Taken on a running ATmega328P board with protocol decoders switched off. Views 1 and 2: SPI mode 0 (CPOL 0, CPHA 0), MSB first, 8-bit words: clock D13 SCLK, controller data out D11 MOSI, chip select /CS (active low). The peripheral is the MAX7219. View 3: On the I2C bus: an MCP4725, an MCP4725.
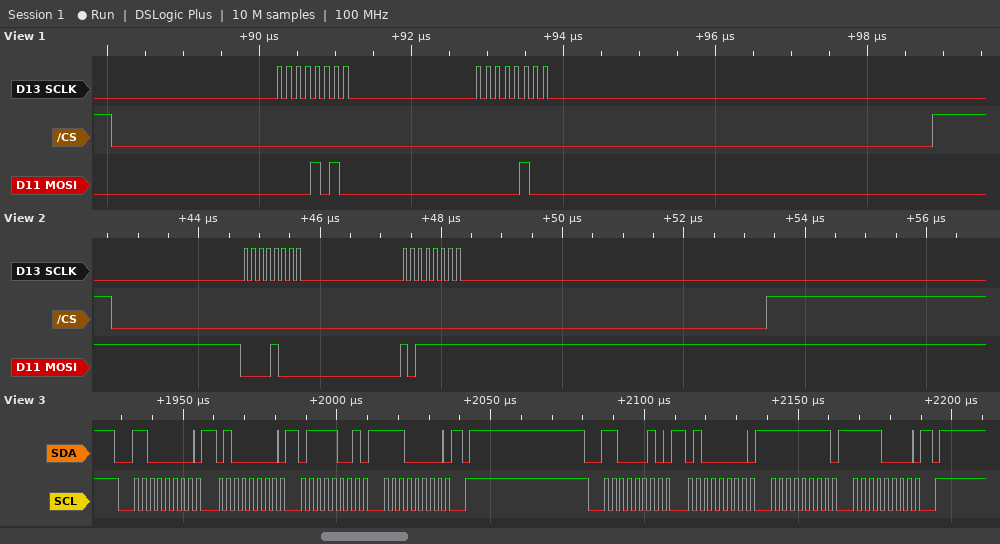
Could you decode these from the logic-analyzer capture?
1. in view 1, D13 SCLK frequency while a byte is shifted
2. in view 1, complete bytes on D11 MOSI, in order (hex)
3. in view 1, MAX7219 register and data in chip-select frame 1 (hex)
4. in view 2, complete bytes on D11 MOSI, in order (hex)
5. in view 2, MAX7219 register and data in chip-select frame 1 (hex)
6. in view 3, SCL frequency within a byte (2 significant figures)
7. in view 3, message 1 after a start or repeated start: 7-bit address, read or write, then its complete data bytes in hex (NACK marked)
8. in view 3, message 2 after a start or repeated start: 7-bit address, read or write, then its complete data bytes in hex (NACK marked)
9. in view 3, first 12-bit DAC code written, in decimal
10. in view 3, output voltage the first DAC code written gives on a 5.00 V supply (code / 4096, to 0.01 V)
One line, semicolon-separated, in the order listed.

8 MHz; 0A 04; register 0xA, data 0x04; 0x08 0xBF; register 0x8, data 0xBF; 400 kHz; 0x60 write: 40 79 E0; 0x61 write: 40 FF F0; 1950; 2.38 V
